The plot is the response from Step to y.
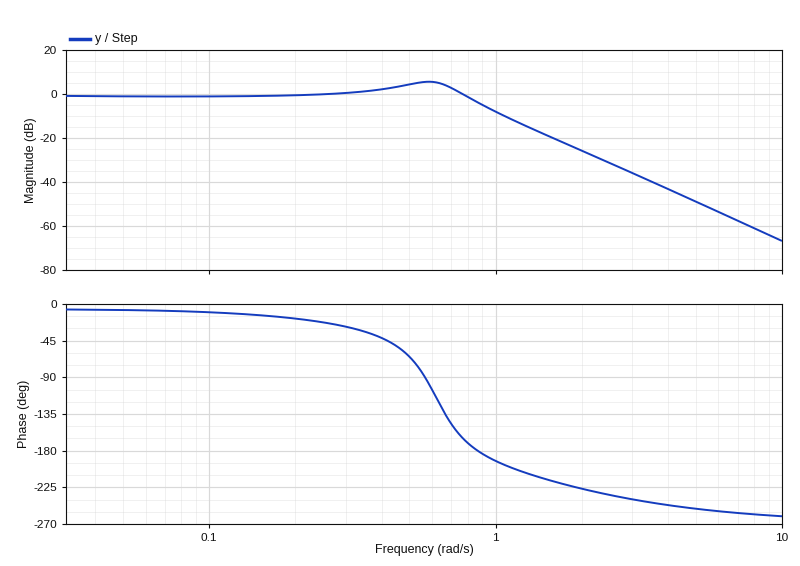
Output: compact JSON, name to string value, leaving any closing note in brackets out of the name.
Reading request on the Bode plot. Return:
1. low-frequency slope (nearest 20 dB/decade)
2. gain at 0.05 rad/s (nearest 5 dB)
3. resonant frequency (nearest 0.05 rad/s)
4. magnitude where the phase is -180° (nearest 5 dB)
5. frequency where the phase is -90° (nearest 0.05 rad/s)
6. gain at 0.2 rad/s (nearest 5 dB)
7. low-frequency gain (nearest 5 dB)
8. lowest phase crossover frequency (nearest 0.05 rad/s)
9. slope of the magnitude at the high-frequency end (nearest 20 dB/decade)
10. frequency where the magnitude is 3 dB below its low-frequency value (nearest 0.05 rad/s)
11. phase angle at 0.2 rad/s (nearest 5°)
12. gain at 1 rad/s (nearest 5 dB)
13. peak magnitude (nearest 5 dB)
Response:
{"low-frequency slope": "0 dB/decade", "gain at 0.05 rad/s": "0 dB", "resonant frequency": "0.60 rad/s", "magnitude where the phase is -180°": "-5 dB", "frequency where the phase is -90°": "0.55 rad/s", "gain at 0.2 rad/s": "0 dB", "low-frequency gain": "0 dB", "lowest phase crossover frequency": "0.85 rad/s", "slope of the magnitude at the high-frequency end": "-60 dB/decade", "frequency where the magnitude is 3 dB below its low-frequency value": "0.85 rad/s", "phase angle at 0.2 rad/s": "-20°", "gain at 1 rad/s": "-10 dB", "peak magnitude": "5 dB"}
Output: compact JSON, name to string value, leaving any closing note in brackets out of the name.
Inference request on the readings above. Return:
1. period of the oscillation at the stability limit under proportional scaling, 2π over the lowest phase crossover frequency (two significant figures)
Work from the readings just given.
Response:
{"period of the oscillation at the stability limit under proportional scaling, 2π over the lowest phase crossover frequency": "7.4 s"}
